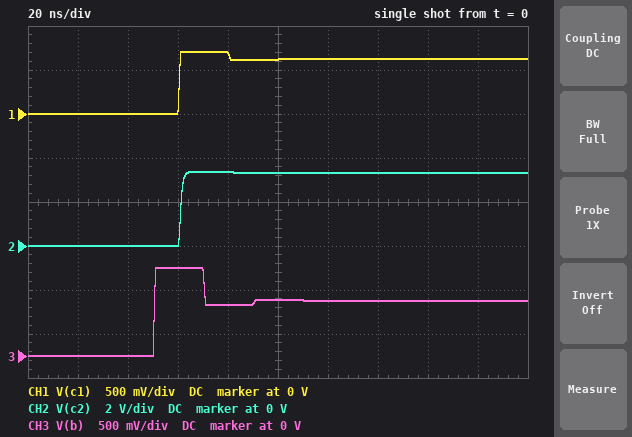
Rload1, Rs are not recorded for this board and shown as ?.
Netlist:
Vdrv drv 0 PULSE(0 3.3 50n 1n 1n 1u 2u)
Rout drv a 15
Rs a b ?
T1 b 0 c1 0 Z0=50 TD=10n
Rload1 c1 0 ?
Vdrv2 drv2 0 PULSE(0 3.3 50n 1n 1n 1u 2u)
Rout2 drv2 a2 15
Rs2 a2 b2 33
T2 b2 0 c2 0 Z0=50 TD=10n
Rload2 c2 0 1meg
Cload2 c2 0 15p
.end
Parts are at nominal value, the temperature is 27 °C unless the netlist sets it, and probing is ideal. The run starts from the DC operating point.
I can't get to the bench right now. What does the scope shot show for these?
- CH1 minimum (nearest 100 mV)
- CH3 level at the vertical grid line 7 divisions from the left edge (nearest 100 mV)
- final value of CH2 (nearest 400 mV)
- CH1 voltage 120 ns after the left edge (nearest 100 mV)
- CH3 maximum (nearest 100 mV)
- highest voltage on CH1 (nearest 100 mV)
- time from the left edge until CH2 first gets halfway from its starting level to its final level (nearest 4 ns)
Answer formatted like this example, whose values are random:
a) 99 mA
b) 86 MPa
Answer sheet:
a) 0 V
b) 600 mV
c) 3.2 V
d) 600 mV
e) 1.0 V
f) 700 mV
g) 60 ns
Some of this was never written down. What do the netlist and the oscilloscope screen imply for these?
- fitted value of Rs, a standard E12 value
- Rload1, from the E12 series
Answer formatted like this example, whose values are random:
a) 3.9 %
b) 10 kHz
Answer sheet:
a) 100 Ω
b) 27 Ω
